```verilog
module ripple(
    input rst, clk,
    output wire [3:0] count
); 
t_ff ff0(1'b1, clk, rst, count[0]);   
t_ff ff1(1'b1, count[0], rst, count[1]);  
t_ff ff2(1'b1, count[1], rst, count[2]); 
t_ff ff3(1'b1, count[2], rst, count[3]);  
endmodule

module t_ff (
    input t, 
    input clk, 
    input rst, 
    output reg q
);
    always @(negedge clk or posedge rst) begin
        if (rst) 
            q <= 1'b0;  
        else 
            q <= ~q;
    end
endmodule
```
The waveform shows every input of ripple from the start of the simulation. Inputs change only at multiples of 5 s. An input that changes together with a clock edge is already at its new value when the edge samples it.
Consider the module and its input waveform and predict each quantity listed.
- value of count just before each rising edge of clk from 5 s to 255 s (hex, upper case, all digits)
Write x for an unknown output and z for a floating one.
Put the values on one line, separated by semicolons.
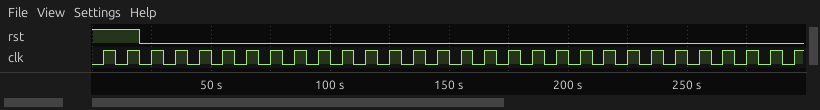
0, 0, 1, 2, 3, 4, 5, 6, 7, 8, 9, A, B, C, D, E, F, 0, 1, 2, 3, 4, 5, 6, 7, 8
